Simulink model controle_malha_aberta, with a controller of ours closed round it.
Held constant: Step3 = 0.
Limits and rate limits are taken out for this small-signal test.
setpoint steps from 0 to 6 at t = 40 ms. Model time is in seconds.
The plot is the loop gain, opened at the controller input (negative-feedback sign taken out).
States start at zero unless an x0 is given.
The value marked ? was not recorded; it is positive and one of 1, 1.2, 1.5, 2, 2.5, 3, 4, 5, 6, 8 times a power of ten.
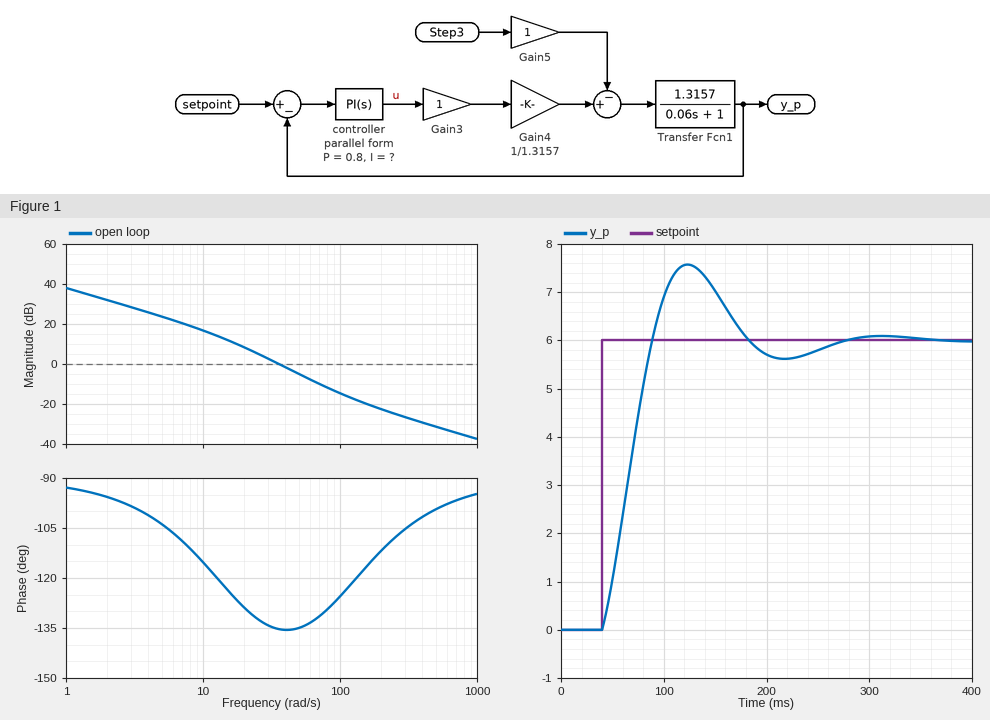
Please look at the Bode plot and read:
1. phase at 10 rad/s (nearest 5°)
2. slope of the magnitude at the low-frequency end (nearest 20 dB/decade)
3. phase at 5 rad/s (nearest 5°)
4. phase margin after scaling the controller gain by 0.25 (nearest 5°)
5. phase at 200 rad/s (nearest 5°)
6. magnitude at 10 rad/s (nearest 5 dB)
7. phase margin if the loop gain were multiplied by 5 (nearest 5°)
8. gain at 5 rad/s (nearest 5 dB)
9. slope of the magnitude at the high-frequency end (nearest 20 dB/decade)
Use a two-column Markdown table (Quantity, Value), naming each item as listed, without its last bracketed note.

| Quantity | Value |
|---|---|
| phase at 10 rad/s | -115° |
| slope of the magnitude at the low-frequency end | -20 dB/decade |
| phase at 5 rad/s | -105° |
| phase margin after scaling the controller gain by 0.25 | 55° |
| phase at 200 rad/s | -110° |
| magnitude at 10 rad/s | 15 dB |
| phase margin if the loop gain were multiplied by 5 | 55° |
| gain at 5 rad/s | 25 dB |
| slope of the magnitude at the high-frequency end | -20 dB/decade |
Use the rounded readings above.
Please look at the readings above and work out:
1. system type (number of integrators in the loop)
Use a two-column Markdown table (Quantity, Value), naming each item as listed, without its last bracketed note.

| Quantity | Value |
|---|---|
| system type | 1 |
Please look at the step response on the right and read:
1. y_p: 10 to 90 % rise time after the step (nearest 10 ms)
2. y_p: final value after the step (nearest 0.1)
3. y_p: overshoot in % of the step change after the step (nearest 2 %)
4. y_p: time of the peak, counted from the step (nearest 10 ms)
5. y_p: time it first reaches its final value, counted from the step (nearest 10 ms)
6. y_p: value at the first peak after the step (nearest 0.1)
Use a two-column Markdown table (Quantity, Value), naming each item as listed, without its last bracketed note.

| Quantity | Value |
|---|---|
| y_p: 10 to 90 % rise time after the step | 40 ms |
| y_p: final value after the step | 6.0 |
| y_p: overshoot in % of the step change after the step | 26 % |
| y_p: time of the peak, counted from the step | 80 ms |
| y_p: time it first reaches its final value, counted from the step | 50 ms |
| y_p: value at the first peak after the step | 7.6 |
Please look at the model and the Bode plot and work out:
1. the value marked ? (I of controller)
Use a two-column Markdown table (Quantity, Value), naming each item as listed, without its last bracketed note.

| Quantity | Value |
|---|---|
| the value marked ? | 80 |
